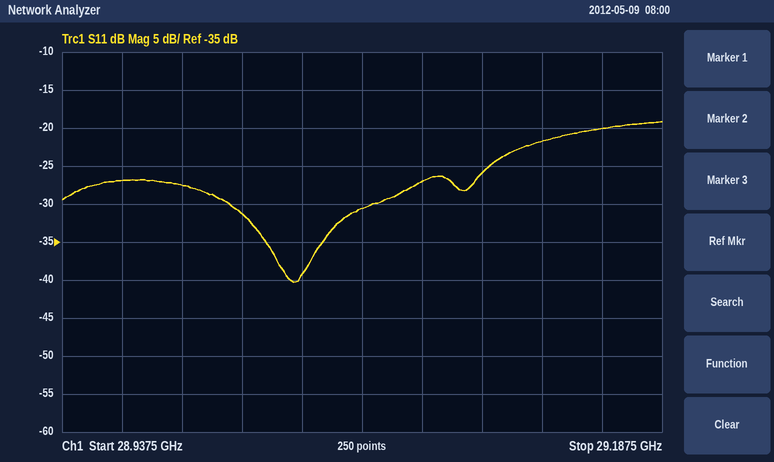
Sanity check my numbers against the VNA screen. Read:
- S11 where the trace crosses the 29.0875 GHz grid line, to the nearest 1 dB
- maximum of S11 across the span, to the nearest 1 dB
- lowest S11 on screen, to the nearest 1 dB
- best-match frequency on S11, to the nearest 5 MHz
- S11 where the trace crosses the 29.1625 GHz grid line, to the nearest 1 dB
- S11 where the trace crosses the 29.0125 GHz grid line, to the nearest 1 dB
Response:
-27 dB
-19 dB
-40 dB
29.035 GHz
-20 dB
-31 dB
